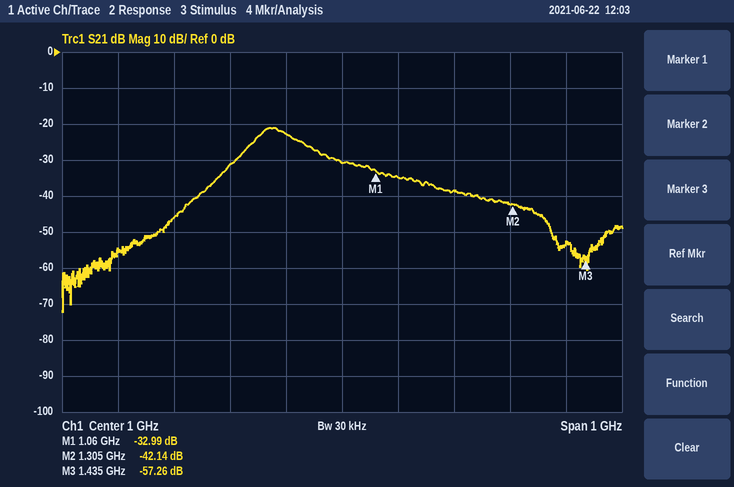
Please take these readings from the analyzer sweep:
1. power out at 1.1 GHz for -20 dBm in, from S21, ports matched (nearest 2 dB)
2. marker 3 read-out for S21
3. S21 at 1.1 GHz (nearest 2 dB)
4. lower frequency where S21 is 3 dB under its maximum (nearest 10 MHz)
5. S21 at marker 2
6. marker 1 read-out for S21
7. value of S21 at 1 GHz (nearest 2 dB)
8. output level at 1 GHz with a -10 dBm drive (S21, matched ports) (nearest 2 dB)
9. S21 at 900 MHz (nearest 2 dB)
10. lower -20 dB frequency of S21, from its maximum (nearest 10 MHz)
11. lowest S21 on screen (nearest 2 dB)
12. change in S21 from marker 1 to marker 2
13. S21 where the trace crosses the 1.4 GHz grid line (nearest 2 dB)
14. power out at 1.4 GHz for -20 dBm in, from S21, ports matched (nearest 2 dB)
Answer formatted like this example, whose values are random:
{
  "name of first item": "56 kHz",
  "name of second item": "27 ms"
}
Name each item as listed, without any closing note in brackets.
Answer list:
{
  "power out at 1.1 GHz for -20 dBm in, from S21, ports matched": "-54 dBm",
  "marker 3 read-out for S21": "-57.26 dB",
  "S21 at 1.1 GHz": "-34 dB",
  "lower frequency where S21 is 3 dB under its maximum": "850 MHz",
  "S21 at marker 2": "-42.14 dB",
  "marker 1 read-out for S21": "-32.99 dB",
  "value of S21 at 1 GHz": "-30 dB",
  "output level at 1 GHz with a -10 dBm drive (S21, matched ports)": "-40 dBm",
  "S21 at 900 MHz": "-22 dB",
  "lower -20 dB frequency of S21, from its maximum": "730 MHz",
  "lowest S21 on screen": "-72 dB",
  "change in S21 from marker 1 to marker 2": "-9.15 dB",
  "S21 where the trace crosses the 1.4 GHz grid line": "-54 dB",
  "power out at 1.4 GHz for -20 dBm in, from S21, ports matched": "-74 dBm"
}
